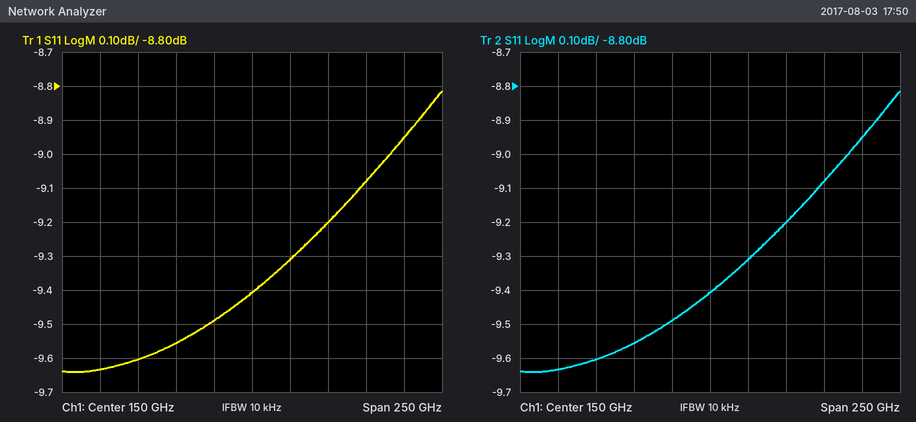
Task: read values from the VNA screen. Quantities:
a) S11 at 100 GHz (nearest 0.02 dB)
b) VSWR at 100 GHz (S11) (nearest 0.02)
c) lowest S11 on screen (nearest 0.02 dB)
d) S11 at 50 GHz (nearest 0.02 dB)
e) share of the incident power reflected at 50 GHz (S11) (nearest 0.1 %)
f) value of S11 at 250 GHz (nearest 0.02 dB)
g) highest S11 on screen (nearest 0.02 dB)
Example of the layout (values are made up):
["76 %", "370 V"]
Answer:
["-9.56 dB", "2.00", "-9.64 dB", "-9.64 dB", "10.9 %", "-8.96 dB", "-8.82 dB"]
